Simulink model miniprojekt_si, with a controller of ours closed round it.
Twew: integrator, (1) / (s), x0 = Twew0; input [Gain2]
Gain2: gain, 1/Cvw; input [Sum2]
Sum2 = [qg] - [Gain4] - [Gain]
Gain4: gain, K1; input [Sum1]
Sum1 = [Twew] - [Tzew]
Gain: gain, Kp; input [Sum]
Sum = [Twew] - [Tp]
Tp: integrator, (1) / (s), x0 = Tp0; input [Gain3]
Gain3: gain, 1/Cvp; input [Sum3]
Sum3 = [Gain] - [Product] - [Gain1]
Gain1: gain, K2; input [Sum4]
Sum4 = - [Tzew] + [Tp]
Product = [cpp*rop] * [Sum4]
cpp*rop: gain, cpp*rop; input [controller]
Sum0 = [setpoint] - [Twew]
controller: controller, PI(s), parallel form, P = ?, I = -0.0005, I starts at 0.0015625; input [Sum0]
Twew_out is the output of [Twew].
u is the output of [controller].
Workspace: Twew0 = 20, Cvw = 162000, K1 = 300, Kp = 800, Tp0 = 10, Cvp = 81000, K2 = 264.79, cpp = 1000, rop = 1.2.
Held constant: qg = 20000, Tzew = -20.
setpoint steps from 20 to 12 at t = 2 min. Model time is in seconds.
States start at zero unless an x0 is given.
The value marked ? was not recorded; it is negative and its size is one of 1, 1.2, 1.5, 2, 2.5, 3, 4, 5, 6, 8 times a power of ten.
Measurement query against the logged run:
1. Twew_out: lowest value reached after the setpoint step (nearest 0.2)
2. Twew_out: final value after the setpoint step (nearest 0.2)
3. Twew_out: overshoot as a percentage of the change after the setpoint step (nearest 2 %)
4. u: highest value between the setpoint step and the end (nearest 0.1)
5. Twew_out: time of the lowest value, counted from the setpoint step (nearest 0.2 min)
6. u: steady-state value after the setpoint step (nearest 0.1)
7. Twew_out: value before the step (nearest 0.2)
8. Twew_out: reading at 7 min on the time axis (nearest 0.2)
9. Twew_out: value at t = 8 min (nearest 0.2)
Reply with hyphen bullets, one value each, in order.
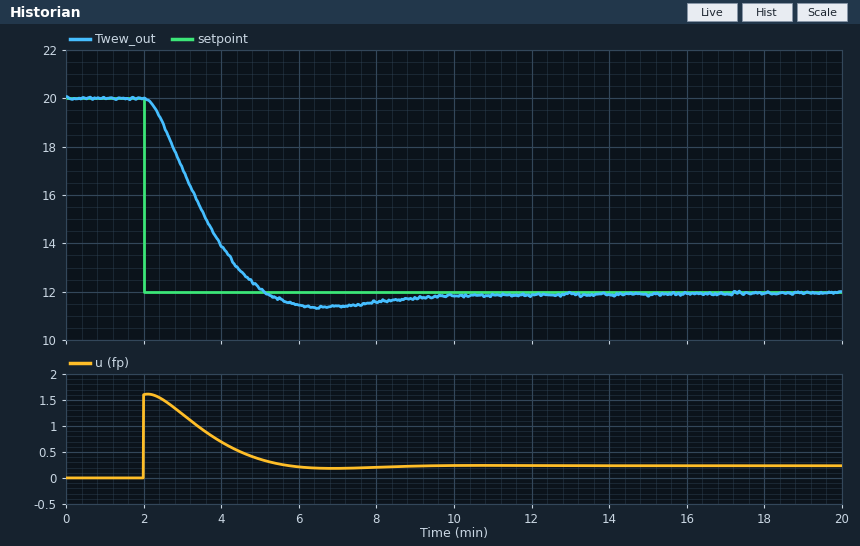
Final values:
- 11.4
- 12.0
- 8 %
- 1.6
- 4.6 min
- 0.2
- 20.0
- 11.4
- 11.6
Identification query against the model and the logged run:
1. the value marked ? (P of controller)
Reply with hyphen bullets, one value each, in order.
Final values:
- -0.2
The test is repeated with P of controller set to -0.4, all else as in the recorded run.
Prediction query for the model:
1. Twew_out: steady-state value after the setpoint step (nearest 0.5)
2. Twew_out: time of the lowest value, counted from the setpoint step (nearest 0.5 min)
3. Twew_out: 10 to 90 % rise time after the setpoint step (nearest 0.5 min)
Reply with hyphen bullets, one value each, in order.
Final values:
- 12.0
- 3.0 min
- 1.5 min
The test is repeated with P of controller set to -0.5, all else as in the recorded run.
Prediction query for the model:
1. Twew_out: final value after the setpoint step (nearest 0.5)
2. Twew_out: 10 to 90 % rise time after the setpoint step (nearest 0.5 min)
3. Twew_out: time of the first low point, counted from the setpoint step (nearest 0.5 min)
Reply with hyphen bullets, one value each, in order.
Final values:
- 12.0
- 1.5 min
- 3.0 min
